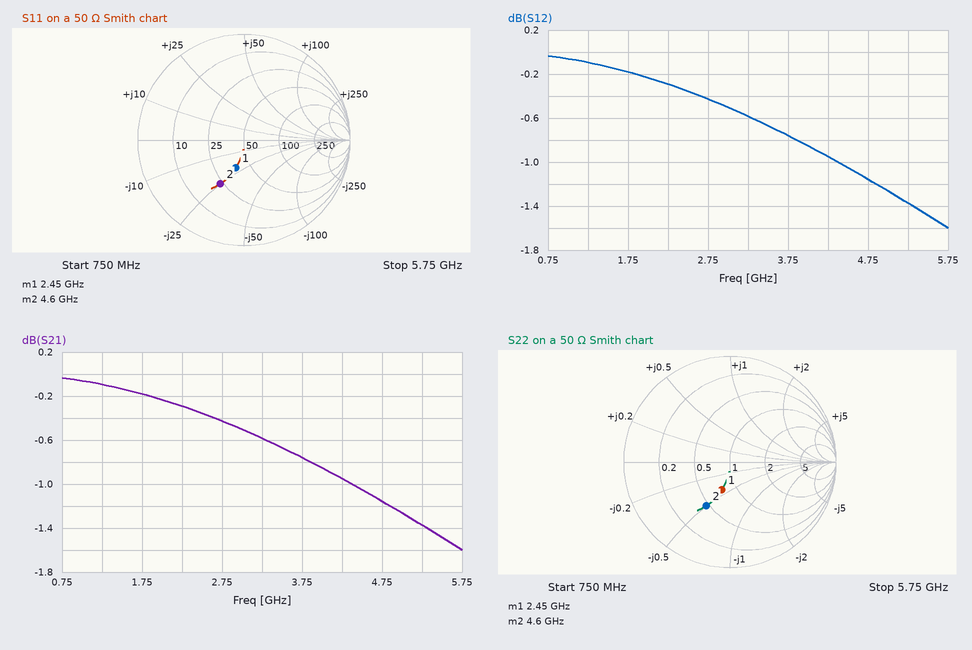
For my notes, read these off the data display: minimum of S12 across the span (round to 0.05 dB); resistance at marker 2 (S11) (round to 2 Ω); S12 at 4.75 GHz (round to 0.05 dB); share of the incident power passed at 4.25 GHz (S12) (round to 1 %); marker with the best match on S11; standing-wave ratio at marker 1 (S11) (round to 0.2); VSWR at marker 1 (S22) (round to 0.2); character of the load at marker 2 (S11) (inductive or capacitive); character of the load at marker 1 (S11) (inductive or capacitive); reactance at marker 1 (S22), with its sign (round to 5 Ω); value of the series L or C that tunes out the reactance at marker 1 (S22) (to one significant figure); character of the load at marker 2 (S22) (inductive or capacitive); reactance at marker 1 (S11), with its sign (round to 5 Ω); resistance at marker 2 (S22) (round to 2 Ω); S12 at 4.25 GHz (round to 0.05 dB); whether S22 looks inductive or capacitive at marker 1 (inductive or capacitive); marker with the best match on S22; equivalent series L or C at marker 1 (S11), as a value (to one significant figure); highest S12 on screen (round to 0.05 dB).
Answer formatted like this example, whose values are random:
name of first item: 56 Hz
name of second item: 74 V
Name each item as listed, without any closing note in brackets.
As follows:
minimum of S12 across the span: -1.60 dB
resistance at marker 2 (S11): 24 Ω
S12 at 4.75 GHz: -1.15 dB
share of the incident power passed at 4.25 GHz (S12): 80 %
marker with the best match on S11: marker 1
standing-wave ratio at marker 1 (S11): 1.8
VSWR at marker 1 (S22): 1.8
character of the load at marker 2 (S11): capacitive
character of the load at marker 1 (S11): capacitive
reactance at marker 1 (S22), with its sign: -20 Ω
value of the series L or C that tunes out the reactance at marker 1 (S22): 1 nH
character of the load at marker 2 (S22): capacitive
reactance at marker 1 (S11), with its sign: -20 Ω
resistance at marker 2 (S22): 24 Ω
S12 at 4.25 GHz: -0.95 dB
whether S22 looks inductive or capacitive at marker 1: capacitive
marker with the best match on S22: marker 1
equivalent series L or C at marker 1 (S11), as a value: 3 pF
highest S12 on screen: -0.05 dB
